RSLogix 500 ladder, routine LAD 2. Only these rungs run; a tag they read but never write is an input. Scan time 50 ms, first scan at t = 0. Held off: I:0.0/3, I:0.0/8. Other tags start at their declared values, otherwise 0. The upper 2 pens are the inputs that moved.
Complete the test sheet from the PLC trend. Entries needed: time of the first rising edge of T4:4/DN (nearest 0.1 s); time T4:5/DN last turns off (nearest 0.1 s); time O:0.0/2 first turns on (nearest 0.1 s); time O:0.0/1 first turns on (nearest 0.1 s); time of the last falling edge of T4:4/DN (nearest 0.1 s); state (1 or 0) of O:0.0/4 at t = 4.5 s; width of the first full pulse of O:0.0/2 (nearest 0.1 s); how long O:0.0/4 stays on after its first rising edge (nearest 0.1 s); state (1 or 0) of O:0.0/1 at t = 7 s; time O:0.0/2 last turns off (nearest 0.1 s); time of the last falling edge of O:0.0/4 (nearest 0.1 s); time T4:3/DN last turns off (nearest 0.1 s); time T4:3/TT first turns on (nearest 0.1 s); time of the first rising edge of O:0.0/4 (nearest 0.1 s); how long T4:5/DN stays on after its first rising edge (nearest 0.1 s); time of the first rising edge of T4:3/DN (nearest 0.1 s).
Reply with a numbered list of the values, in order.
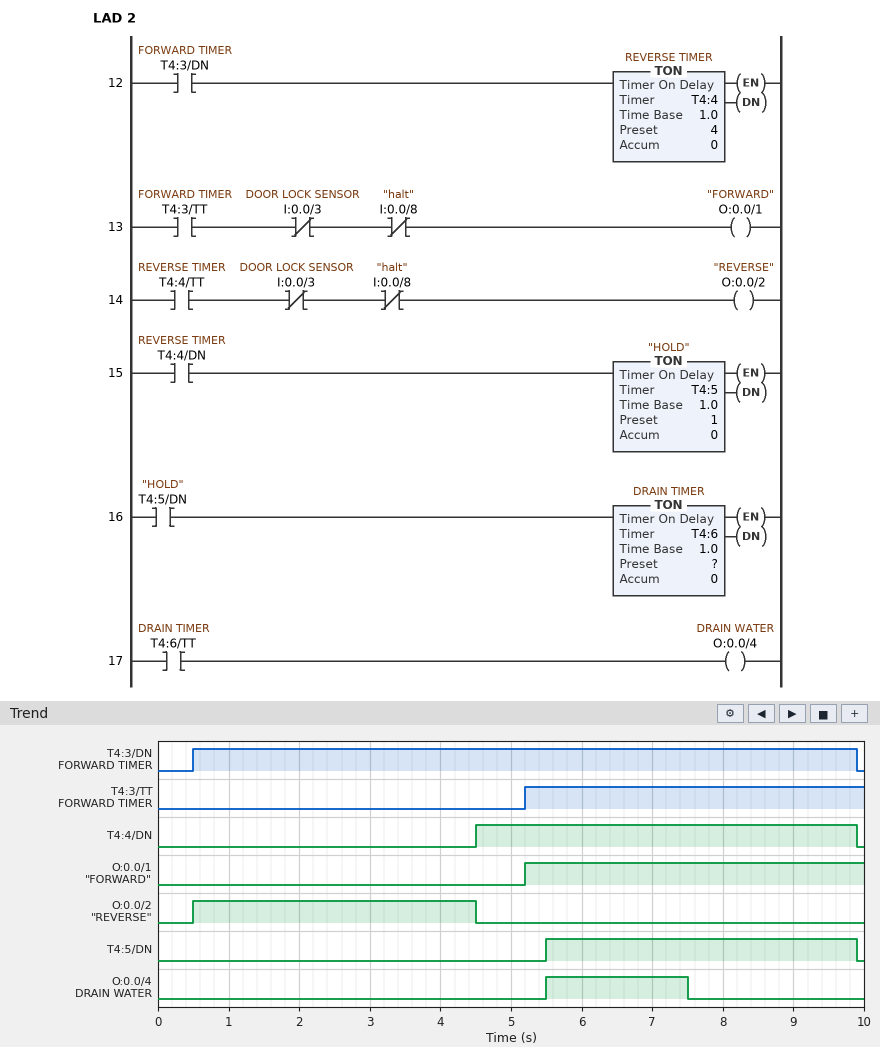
1. 4.5 s
2. 9.9 s
3. 0.5 s
4. 5.2 s
5. 9.9 s
6. 0
7. 4.0 s
8. 2.0 s
9. 1
10. 4.5 s
11. 7.5 s
12. 9.9 s
13. 5.2 s
14. 5.5 s
15. 4.4 s
16. 0.5 s
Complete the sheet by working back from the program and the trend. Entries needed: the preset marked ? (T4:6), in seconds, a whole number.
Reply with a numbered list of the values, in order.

1. 2 s
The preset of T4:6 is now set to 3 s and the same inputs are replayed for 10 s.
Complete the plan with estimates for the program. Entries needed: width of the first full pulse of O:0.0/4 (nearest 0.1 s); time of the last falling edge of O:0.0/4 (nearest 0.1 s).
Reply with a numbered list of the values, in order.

1. 3.0 s
2. 8.5 s
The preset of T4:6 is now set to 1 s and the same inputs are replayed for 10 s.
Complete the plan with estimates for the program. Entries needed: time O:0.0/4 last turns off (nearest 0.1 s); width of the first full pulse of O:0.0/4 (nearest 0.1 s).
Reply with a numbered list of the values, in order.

1. 6.5 s
2. 1.0 s
